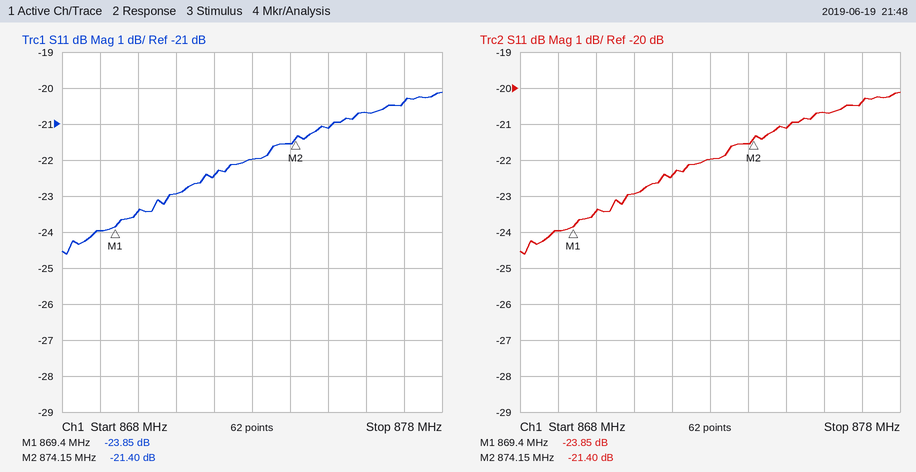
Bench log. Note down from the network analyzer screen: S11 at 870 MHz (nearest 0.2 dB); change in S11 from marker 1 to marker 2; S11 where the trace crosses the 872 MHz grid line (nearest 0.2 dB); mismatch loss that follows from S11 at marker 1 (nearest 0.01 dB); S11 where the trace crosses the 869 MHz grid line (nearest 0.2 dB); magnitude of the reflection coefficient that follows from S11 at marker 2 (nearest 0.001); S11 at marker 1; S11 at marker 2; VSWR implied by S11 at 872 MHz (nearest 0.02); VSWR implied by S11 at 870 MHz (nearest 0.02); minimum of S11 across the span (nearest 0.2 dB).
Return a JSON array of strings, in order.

["-23.4 dB", "2.45 dB", "-22.4 dB", "0.02 dB", "-24.0 dB", "0.085", "-23.85 dB", "-21.40 dB", "1.16", "1.14", "-24.6 dB"]
